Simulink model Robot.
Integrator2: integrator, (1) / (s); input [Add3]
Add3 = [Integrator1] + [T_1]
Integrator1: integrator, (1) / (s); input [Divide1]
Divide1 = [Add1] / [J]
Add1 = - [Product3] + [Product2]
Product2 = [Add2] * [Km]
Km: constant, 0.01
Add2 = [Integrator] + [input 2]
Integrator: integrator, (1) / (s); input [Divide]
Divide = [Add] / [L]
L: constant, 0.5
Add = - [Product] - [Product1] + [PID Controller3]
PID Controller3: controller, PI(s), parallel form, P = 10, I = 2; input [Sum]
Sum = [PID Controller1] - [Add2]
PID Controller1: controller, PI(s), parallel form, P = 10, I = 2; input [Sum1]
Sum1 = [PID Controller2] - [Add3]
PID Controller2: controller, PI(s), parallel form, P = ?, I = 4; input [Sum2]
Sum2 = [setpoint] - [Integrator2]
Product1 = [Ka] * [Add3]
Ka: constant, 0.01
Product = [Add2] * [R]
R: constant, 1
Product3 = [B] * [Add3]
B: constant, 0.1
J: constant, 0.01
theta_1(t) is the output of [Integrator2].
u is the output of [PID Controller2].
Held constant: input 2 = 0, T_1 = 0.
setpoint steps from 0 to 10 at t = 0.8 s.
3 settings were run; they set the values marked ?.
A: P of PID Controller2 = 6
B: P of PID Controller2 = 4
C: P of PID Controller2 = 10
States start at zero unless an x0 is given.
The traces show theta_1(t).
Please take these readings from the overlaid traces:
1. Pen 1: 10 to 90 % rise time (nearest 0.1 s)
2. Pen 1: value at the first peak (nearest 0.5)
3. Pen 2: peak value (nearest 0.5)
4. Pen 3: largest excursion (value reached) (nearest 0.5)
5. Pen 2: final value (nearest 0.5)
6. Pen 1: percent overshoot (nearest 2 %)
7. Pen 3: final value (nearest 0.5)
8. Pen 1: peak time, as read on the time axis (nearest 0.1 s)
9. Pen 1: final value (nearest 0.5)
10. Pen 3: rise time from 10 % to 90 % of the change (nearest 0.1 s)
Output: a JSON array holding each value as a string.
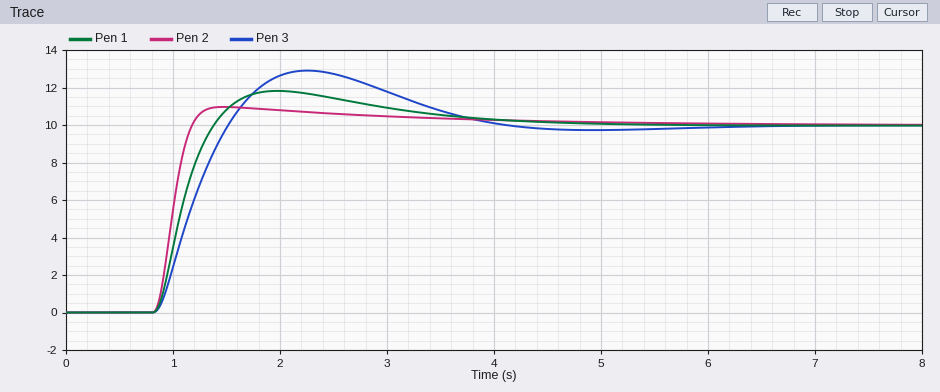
["0.4 s", "12.0", "11.0", "13.0", "10.0", "18 %", "10.0", "2.0 s", "10.0", "0.5 s"]
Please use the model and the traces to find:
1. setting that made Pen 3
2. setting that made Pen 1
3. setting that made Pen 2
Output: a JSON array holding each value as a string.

["B", "A", "C"]
